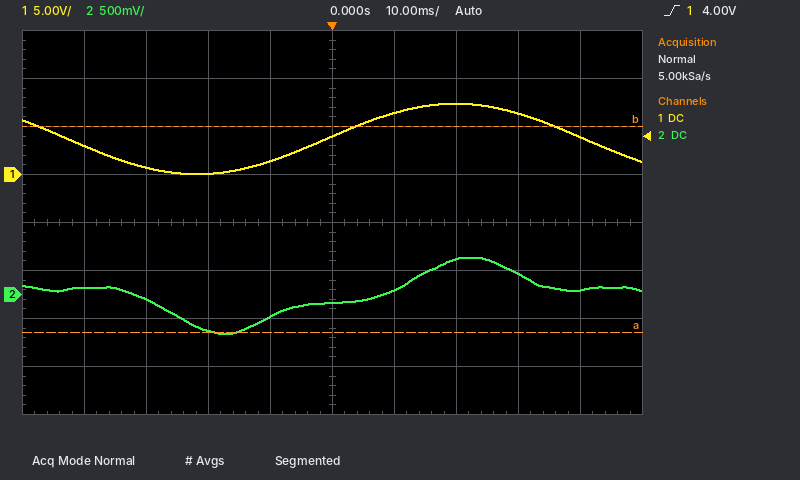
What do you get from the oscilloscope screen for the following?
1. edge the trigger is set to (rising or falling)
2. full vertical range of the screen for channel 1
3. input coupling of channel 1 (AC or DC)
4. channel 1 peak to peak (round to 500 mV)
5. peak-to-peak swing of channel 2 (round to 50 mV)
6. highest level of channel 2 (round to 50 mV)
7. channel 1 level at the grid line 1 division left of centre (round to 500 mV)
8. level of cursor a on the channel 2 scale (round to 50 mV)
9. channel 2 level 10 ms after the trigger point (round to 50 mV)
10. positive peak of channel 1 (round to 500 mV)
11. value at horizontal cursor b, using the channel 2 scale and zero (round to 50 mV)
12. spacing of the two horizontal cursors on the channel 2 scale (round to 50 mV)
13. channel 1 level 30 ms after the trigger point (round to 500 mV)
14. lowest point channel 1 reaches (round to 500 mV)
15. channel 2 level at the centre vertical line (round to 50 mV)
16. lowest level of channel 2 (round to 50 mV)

rising
40 V
DC
7.5 V
800 mV
400 mV
1.5 V
-400 mV
50 mV
7.5 V
1.75 V
2.15 V
6.5 V
0.0 V
-100 mV
-400 mV
